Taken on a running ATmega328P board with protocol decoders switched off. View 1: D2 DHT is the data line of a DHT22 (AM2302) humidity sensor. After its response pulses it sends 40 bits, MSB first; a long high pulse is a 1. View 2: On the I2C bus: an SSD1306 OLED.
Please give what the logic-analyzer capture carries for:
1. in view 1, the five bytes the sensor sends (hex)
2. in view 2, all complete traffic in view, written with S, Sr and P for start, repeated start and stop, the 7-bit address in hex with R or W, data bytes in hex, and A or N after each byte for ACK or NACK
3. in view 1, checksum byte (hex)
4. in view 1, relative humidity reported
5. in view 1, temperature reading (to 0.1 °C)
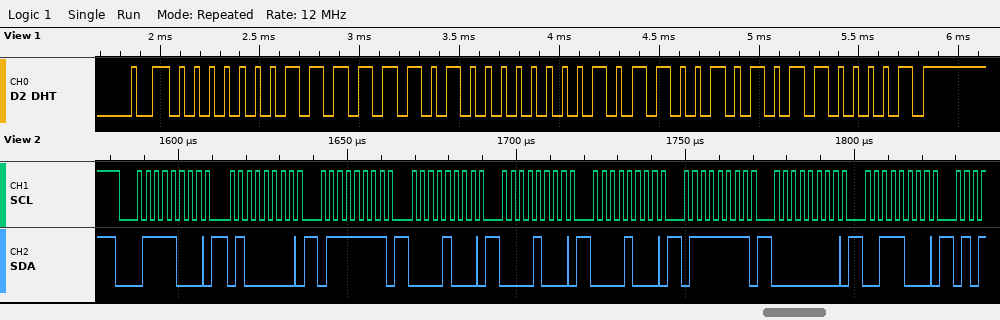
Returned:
01 FA 01 65 61
S 3CW A 40 A 7F A 08 A 08 A 08 A 7F A 00 A 38 A
0x61
50.6 %
35.7 °C
